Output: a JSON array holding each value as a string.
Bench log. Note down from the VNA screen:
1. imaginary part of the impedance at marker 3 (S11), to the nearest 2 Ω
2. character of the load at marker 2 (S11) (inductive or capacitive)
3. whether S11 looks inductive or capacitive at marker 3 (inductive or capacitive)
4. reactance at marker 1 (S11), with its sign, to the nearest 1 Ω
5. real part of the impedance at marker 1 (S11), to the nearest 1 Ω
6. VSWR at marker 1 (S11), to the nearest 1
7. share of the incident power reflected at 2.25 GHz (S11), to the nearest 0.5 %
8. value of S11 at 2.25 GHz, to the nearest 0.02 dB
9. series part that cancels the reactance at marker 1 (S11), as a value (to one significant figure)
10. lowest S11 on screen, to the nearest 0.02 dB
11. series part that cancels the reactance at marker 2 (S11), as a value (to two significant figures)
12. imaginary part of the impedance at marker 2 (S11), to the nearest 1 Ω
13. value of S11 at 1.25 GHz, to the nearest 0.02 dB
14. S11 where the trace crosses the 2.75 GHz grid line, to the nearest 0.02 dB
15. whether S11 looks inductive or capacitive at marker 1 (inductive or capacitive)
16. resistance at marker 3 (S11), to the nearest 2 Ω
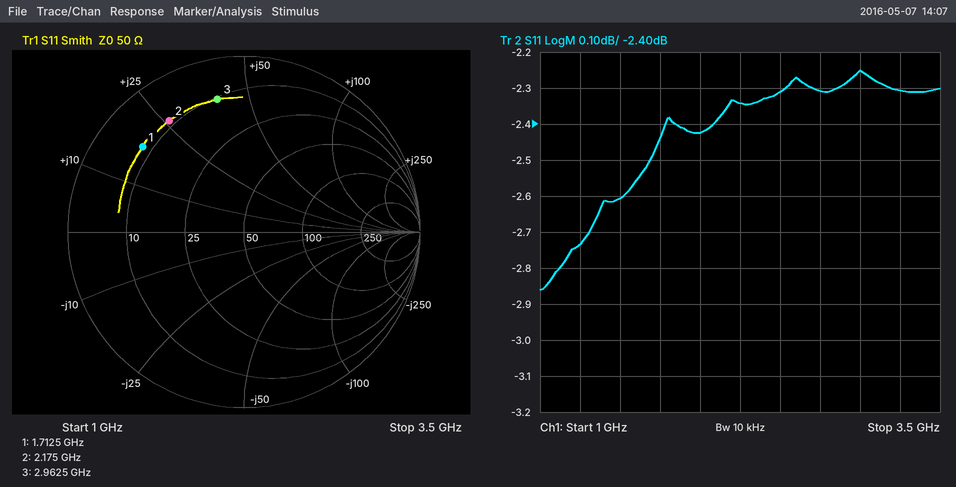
["+40 Ω", "inductive", "inductive", "+18 Ω", "8 Ω", "7", "58.5 %", "-2.34 dB", "5 pF", "-2.86 dB", "2.8 pF", "+26 Ω", "-2.74 dB", "-2.30 dB", "inductive", "10 Ω"]
